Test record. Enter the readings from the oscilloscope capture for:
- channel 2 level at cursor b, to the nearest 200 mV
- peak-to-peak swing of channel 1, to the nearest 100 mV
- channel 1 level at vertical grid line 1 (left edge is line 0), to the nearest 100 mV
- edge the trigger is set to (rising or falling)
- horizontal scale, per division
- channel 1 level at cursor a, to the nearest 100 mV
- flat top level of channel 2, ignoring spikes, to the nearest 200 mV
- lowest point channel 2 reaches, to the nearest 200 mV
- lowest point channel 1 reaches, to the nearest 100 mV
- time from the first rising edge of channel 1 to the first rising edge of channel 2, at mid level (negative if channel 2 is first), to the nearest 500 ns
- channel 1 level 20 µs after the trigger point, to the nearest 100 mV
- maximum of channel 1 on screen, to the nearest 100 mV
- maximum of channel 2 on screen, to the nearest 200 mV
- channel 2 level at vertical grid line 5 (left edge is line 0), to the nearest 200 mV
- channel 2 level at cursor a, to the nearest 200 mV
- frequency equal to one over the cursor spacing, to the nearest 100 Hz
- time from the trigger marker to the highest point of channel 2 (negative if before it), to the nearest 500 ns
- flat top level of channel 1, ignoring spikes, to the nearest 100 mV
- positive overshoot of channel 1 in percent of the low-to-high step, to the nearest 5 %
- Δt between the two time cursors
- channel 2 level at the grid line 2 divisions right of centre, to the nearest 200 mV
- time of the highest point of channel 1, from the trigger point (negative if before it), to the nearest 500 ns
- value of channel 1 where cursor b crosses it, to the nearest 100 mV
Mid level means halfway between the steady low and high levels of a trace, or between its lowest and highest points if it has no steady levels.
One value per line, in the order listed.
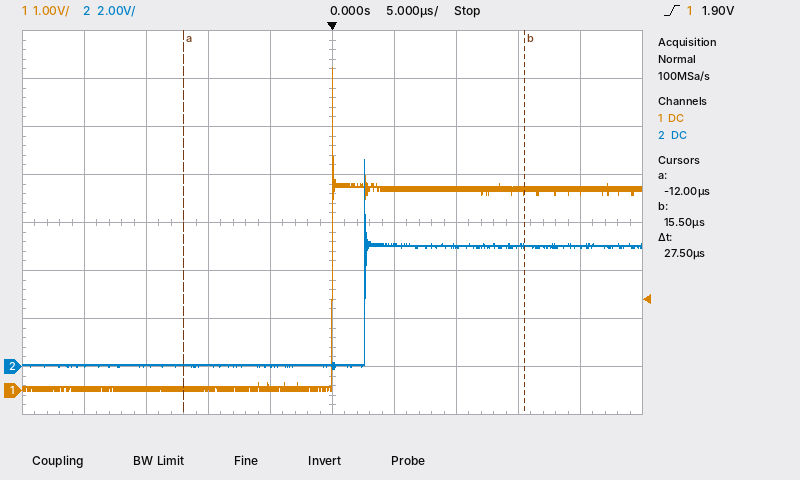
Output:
5.0 V
6.7 V
0.0 V
rising
5 µs
0.0 V
5.0 V
0.0 V
0.0 V
+2.5 µs
4.2 V
6.7 V
8.6 V
0.0 V
0.0 V
36.4 kHz
+2.5 µs
4.2 V
60 %
27.5 µs
5.0 V
0.0 µs
4.2 V
